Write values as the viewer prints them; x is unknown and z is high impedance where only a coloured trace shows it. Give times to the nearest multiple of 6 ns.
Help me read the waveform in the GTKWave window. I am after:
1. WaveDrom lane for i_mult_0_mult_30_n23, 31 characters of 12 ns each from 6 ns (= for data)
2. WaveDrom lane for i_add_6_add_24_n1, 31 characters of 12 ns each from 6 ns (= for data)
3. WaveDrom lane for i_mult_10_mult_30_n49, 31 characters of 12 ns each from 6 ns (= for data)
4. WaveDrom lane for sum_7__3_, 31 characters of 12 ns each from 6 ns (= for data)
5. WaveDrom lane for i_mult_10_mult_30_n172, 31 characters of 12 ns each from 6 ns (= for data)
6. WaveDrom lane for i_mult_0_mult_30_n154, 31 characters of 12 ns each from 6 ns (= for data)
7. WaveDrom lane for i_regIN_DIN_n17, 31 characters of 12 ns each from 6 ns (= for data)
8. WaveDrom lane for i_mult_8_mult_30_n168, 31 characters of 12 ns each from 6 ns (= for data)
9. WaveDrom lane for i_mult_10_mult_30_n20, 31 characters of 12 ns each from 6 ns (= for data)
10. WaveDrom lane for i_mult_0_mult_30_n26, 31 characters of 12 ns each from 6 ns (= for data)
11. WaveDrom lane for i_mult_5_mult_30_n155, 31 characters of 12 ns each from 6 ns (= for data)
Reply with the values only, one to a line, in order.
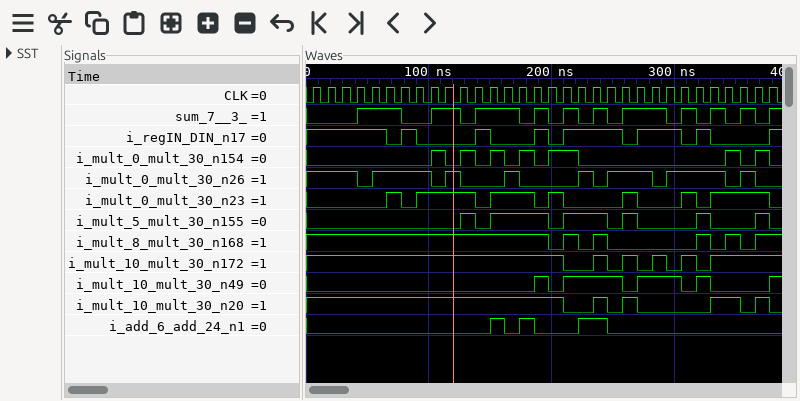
{name: 'i_mult_0_mult_30_n23', wave: '0....101...01..010...10..101...'}
{name: 'i_add_6_add_24_n1', wave: '0...........1010..1.0..........'}
{name: 'i_mult_10_mult_30_n49', wave: '0..............101...01..010...'}
{name: 'sum_7__3_', wave: '0..1..0.1.01..01010101..0101010'}
{name: 'i_mult_10_mult_30_n172', wave: '1................0.101010101...'}
{name: 'i_mult_0_mult_30_n154', wave: '0.......101010101.0.........101'}
{name: 'i_regIN_DIN_n17', wave: '1....010...10..101...01..010...'}
{name: 'i_mult_8_mult_30_n168', wave: '1...............01010.....10101'}
{name: 'i_mult_10_mult_30_n20', wave: '1................0.1010....1.01'}
{name: 'i_mult_0_mult_30_n26', wave: '1..01...010..10...101..01...010'}
{name: 'i_mult_5_mult_30_n155', wave: '0.........101...01..010...10..1'}
